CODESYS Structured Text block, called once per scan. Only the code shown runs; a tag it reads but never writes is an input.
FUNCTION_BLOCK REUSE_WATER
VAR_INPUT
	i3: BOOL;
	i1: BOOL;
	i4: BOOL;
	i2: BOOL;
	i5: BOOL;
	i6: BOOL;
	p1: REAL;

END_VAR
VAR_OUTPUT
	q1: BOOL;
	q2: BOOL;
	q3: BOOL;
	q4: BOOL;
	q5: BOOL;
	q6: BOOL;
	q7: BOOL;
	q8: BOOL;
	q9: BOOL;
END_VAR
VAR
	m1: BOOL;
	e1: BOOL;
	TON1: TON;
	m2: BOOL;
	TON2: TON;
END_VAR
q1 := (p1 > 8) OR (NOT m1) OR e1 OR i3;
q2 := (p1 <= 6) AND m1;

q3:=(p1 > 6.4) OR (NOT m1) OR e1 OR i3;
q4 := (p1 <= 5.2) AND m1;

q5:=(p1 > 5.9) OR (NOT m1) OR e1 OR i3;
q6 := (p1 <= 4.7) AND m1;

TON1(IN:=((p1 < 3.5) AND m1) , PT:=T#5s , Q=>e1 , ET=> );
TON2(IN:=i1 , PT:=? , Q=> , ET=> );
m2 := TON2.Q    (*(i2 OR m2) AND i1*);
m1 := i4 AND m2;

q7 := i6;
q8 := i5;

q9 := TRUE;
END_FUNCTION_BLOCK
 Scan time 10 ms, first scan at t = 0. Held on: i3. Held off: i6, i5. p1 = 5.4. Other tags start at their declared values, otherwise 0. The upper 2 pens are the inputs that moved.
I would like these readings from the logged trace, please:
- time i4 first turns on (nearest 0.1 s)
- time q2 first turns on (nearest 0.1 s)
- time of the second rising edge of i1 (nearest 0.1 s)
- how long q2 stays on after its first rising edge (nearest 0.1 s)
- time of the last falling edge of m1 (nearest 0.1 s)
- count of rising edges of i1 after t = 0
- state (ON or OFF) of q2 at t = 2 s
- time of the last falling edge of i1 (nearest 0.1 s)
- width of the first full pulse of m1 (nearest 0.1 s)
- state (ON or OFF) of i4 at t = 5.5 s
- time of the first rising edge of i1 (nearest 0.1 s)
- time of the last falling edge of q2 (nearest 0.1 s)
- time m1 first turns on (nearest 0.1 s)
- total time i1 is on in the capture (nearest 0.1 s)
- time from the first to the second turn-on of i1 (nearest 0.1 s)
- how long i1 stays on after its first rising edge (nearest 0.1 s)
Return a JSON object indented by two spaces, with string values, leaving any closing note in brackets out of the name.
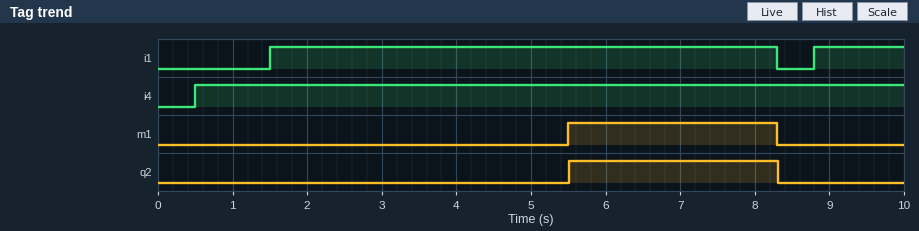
{
  "time i4 first turns on": "0.5 s",
  "time q2 first turns on": "5.5 s",
  "time of the second rising edge of i1": "8.8 s",
  "how long q2 stays on after its first rising edge": "2.8 s",
  "time of the last falling edge of m1": "8.3 s",
  "count of rising edges of i1 after t = 0": "2",
  "state (ON or OFF) of q2 at t = 2 s": "OFF",
  "time of the last falling edge of i1": "8.3 s",
  "width of the first full pulse of m1": "2.8 s",
  "state (ON or OFF) of i4 at t = 5.5 s": "ON",
  "time of the first rising edge of i1": "1.5 s",
  "time of the last falling edge of q2": "8.3 s",
  "time m1 first turns on": "5.5 s",
  "total time i1 is on in the capture": "8.0 s",
  "time from the first to the second turn-on of i1": "7.3 s",
  "how long i1 stays on after its first rising edge": "6.8 s"
}
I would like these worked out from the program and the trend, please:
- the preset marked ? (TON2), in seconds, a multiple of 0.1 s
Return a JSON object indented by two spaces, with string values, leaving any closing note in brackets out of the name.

{
  "the preset marked ? (TON2), in seconds, a multiple of 0.1 s": "4.0 s"
}
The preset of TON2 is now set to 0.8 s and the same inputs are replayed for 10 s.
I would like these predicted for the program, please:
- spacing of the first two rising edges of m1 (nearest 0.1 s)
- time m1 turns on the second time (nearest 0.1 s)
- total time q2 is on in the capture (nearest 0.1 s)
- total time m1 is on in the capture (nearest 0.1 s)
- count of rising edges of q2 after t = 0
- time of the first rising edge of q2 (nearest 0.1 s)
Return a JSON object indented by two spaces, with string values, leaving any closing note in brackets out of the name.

{
  "spacing of the first two rising edges of m1": "7.3 s",
  "time m1 turns on the second time": "9.6 s",
  "total time q2 is on in the capture": "6.4 s",
  "total time m1 is on in the capture": "6.4 s",
  "count of rising edges of q2 after t = 0": "2",
  "time of the first rising edge of q2": "2.3 s"
}
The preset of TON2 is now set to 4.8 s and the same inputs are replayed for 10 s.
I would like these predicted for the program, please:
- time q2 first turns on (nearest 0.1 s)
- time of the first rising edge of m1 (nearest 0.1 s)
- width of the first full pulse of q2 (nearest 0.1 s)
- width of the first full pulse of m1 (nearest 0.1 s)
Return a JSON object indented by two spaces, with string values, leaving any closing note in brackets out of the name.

{
  "time q2 first turns on": "6.3 s",
  "time of the first rising edge of m1": "6.3 s",
  "width of the first full pulse of q2": "2.0 s",
  "width of the first full pulse of m1": "2.0 s"
}
